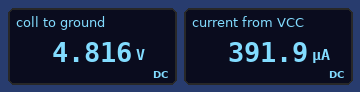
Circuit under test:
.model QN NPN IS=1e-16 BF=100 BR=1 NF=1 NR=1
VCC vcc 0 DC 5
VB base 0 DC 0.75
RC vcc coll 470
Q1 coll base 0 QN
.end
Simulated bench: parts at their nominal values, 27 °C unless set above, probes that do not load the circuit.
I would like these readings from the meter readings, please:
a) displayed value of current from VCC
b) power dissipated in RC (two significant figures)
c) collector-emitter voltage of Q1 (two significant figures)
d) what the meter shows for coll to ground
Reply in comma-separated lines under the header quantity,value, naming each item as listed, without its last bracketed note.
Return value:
quantity,value
displayed value of current from VCC,391.9 µA
power dissipated in RC,72 µW
collector-emitter voltage of Q1,4.8 V
what the meter shows for coll to ground,4.816 V
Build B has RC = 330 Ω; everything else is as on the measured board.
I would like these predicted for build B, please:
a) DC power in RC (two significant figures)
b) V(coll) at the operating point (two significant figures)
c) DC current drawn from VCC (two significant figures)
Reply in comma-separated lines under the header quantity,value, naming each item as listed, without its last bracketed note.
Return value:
quantity,value
DC power in RC,51 µW
V(coll) at the operating point,4.9 V
DC current drawn from VCC,390 µA
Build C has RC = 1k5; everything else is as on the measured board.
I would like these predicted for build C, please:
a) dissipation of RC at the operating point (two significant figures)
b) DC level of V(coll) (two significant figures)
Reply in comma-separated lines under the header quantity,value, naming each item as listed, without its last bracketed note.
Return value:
quantity,value
dissipation of RC at the operating point,230 µW
DC level of V(coll),4.4 V
